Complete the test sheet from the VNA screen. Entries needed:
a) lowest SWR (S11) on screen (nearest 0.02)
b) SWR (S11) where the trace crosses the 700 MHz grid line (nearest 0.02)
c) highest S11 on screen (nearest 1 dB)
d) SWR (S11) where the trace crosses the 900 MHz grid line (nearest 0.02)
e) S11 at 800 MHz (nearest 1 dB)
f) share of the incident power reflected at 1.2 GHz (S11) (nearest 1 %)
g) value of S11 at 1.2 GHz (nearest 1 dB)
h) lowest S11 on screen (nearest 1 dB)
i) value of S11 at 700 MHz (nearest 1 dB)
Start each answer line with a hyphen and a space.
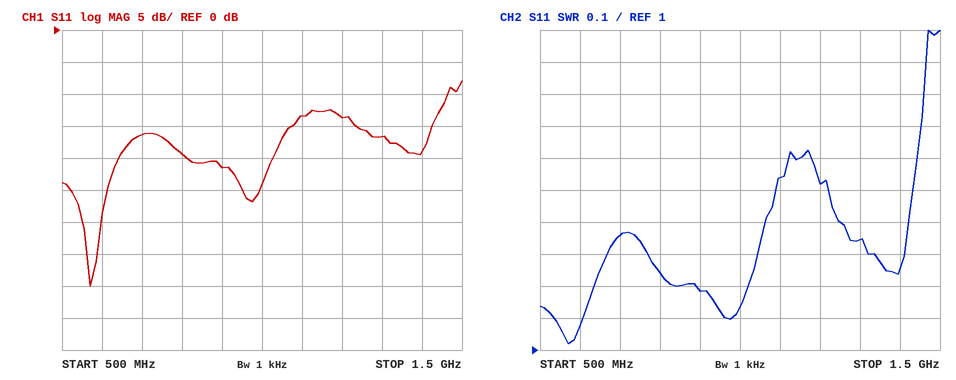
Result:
- 1.02
- 1.36
- -8 dB
- 1.18
- -19 dB
- 4 %
- -14 dB
- -40 dB
- -16 dB
